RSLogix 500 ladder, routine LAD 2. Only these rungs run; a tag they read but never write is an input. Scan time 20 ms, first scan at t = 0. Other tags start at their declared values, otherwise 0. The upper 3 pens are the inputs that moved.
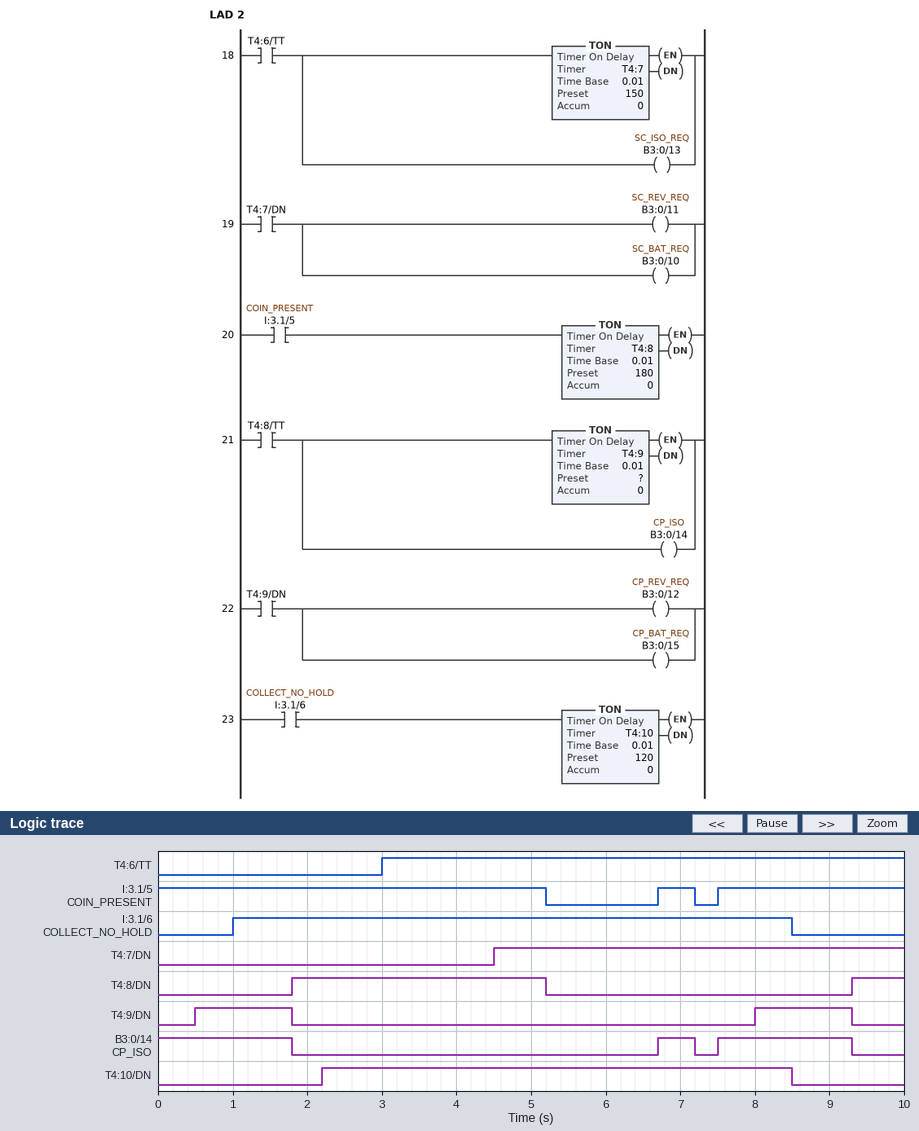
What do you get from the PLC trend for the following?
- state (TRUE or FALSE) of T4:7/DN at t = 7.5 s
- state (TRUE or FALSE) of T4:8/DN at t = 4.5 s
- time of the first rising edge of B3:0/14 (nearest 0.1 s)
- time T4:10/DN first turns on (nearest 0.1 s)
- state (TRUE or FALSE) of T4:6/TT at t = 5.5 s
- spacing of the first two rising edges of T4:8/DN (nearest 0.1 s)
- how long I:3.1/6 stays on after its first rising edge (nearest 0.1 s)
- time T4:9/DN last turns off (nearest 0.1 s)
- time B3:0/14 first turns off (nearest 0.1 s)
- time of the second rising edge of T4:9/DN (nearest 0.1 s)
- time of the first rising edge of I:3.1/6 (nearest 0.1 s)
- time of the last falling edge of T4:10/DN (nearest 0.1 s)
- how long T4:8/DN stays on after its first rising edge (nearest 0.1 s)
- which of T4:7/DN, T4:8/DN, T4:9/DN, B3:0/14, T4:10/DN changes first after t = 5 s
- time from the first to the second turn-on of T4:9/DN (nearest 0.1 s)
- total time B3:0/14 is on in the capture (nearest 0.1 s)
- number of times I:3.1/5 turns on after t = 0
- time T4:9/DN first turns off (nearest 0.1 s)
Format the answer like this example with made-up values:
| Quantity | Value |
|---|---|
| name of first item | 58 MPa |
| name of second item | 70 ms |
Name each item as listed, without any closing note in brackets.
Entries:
| Quantity | Value |
|---|---|
| state (TRUE or FALSE) of T4:7/DN at t = 7.5 s | TRUE |
| state (TRUE or FALSE) of T4:8/DN at t = 4.5 s | TRUE |
| time of the first rising edge of B3:0/14 | 6.7 s |
| time T4:10/DN first turns on | 2.2 s |
| state (TRUE or FALSE) of T4:6/TT at t = 5.5 s | TRUE |
| spacing of the first two rising edges of T4:8/DN | 7.5 s |
| how long I:3.1/6 stays on after its first rising edge | 7.5 s |
| time T4:9/DN last turns off | 9.3 s |
| time B3:0/14 first turns off | 1.8 s |
| time of the second rising edge of T4:9/DN | 8.0 s |
| time of the first rising edge of I:3.1/6 | 1.0 s |
| time of the last falling edge of T4:10/DN | 8.5 s |
| how long T4:8/DN stays on after its first rising edge | 3.4 s |
| which of T4:7/DN, T4:8/DN, T4:9/DN, B3:0/14, T4:10/DN changes first after t = 5 s | T4:8/DN |
| time from the first to the second turn-on of T4:9/DN | 7.5 s |
| total time B3:0/14 is on in the capture | 4.1 s |
| number of times I:3.1/5 turns on after t = 0 | 2 |
| time T4:9/DN first turns off | 1.8 s |
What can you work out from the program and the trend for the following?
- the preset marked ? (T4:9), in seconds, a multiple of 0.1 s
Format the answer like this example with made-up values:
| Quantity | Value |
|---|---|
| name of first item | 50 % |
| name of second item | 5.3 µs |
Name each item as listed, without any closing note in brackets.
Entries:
| Quantity | Value |
|---|---|
| the preset marked ? (T4:9), in seconds, a multiple of 0.1 s | 0.5 s |
